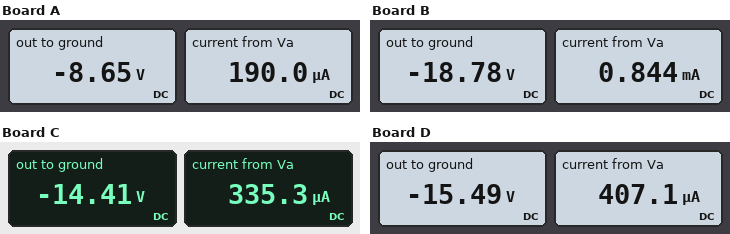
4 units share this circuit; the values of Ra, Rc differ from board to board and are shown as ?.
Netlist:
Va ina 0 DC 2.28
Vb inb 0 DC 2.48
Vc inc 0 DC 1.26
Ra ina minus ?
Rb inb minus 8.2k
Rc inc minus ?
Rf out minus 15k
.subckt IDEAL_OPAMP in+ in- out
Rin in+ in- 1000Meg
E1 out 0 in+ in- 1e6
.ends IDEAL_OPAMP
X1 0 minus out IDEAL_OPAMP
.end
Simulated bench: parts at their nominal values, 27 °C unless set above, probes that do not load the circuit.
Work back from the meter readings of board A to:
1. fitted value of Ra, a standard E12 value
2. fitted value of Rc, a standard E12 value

12 kΩ
15 kΩ
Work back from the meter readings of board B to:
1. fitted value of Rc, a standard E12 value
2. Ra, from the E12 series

12 kΩ
2.7 kΩ
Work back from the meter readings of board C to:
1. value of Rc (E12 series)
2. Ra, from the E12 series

3.9 kΩ
6.8 kΩ
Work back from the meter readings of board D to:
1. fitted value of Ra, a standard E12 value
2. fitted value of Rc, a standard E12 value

5.6 kΩ
3.9 kΩ
